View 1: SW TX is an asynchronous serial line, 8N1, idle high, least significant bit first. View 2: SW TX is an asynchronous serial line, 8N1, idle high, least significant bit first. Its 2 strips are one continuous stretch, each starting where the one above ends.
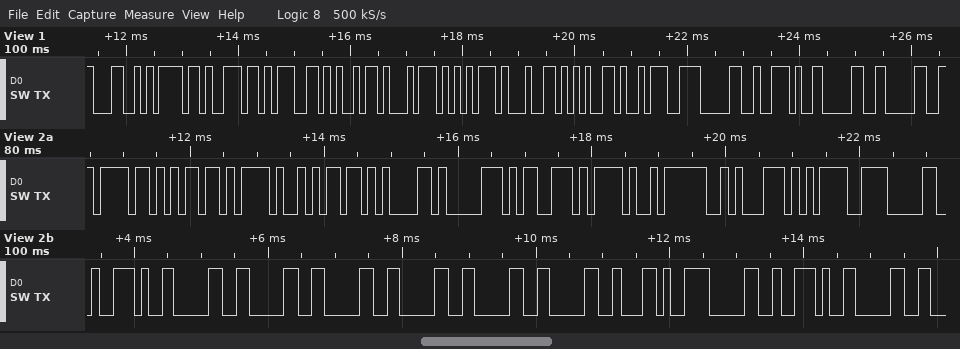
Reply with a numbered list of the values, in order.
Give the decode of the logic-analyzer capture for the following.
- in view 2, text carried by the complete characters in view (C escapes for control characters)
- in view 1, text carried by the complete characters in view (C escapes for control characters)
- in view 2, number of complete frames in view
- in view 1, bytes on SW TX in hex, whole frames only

1. "om/maps/?q=0.000000,0.0"
2. "Longitude:0.00"
3. 23
4. 4C 6F 6E 67 69 74 75 64 65 3A 30 2E 30 30
